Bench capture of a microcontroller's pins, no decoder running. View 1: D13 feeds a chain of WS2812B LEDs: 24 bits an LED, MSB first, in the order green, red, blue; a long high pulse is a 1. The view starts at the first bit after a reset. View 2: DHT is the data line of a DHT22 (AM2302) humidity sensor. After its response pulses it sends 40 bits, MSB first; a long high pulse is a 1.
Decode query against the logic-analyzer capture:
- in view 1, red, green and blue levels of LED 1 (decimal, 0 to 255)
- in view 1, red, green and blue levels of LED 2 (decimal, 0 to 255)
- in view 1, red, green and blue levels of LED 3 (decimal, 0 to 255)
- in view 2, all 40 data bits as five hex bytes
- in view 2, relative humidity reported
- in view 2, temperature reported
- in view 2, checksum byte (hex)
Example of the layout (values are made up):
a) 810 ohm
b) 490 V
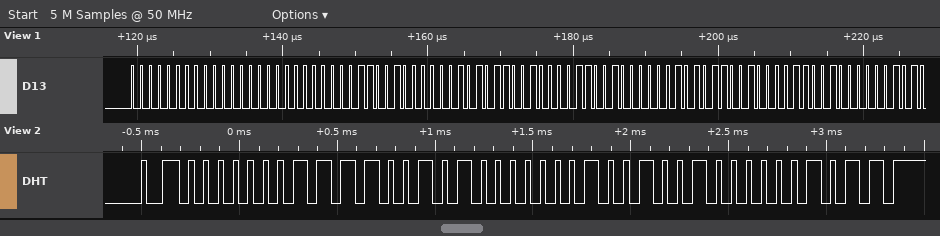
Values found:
a) 0, 0, 0
b) 10, 100, 200
c) 10, 100, 200
d) 01 E5 01 24 0B
e) 48.5 %
f) 29.2 °C
g) 0x0B
